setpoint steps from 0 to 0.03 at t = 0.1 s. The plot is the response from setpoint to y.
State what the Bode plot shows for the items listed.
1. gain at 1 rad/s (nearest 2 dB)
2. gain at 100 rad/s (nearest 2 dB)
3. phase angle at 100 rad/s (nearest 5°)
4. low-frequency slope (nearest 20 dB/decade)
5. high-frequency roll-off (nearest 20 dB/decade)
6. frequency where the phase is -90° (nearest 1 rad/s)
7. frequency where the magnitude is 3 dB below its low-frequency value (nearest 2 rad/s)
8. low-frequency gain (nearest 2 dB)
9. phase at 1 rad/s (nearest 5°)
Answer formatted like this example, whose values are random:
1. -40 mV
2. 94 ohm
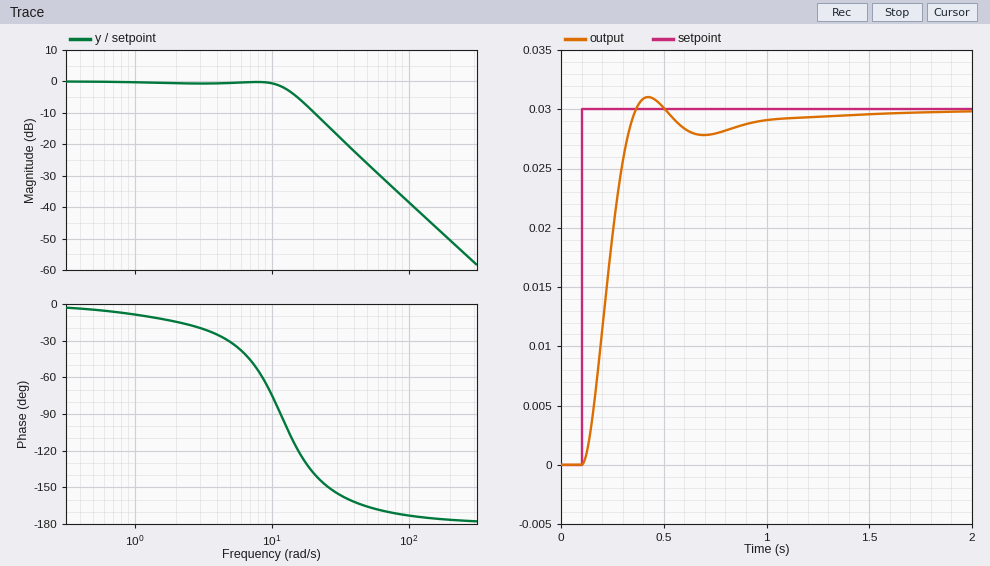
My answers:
1. 0 dB
2. -38 dB
3. -175°
4. 0 dB/decade
5. -40 dB/decade
6. 12 rad/s
7. 14 rad/s
8. 0 dB
9. -10°
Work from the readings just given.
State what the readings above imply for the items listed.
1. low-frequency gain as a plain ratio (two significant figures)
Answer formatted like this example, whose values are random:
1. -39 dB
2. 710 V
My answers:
1. 1.0
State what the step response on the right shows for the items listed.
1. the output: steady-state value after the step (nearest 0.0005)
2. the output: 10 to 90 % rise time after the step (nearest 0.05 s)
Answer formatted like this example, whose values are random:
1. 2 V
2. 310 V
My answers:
1. 0.0300
2. 0.15 s
